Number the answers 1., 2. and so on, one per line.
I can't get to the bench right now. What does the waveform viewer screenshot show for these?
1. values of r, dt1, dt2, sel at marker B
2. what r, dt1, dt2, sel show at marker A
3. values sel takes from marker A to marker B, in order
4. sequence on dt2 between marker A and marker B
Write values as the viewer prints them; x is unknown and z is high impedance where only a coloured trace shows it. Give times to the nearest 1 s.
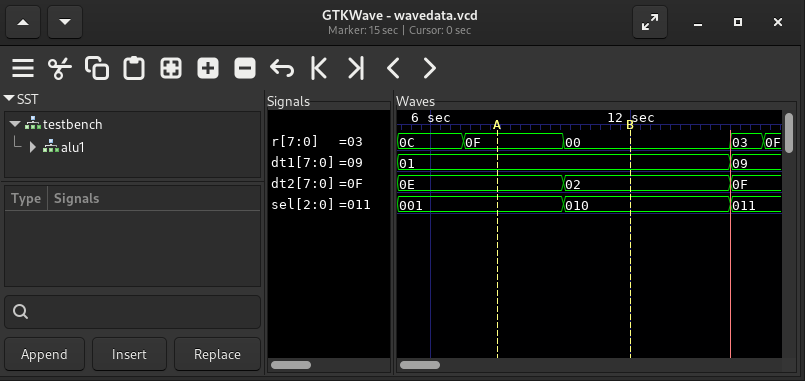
1. r=00, dt1=01, dt2=02, sel=010
2. r=0F, dt1=01, dt2=0E, sel=001
3. 001, 010
4. 0E, 02
